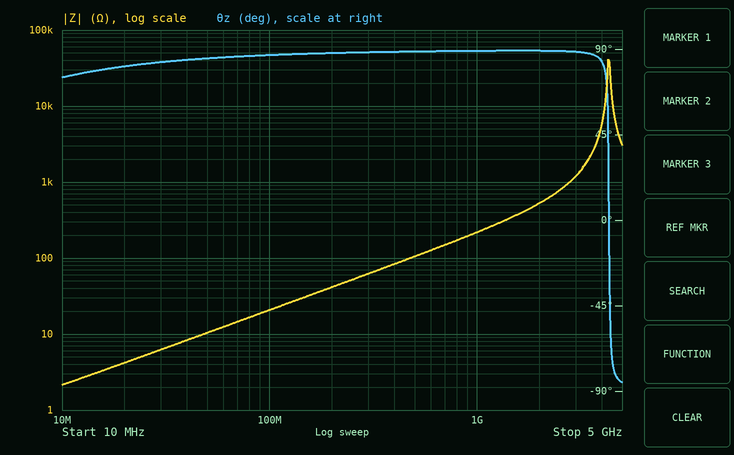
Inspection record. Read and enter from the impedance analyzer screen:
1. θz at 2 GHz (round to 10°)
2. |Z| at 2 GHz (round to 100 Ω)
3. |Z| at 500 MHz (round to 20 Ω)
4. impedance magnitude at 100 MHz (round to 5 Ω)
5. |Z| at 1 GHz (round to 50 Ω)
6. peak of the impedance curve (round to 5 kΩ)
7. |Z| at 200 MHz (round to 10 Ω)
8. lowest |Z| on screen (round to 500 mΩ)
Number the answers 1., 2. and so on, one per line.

1. 90°
2. 500 Ω
3. 100 Ω
4. 20 Ω
5. 200 Ω
6. 40 kΩ
7. 40 Ω
8. 2.0 Ω
